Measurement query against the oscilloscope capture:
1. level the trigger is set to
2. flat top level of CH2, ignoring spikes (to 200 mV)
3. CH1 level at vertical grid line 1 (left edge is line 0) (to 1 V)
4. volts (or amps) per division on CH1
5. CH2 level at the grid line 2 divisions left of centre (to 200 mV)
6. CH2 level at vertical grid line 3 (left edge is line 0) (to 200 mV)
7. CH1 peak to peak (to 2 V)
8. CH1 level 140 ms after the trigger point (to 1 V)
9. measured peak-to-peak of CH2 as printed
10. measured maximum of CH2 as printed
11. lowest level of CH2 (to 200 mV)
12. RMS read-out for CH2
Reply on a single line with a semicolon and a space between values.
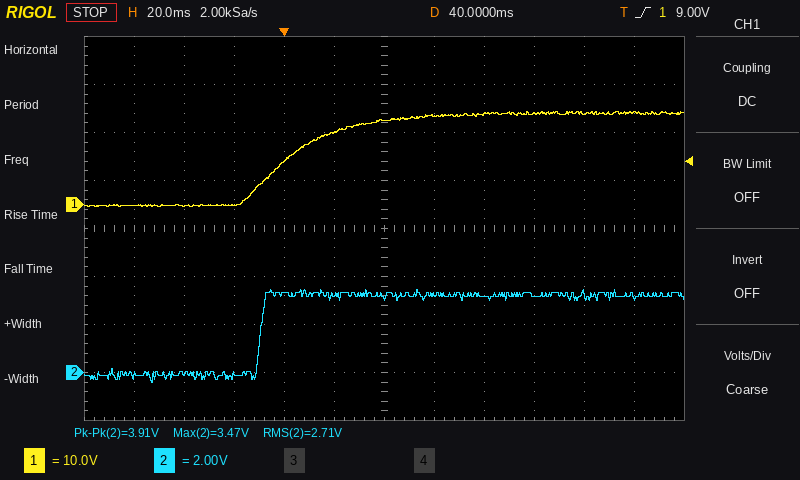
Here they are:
9.00 V; 3.2 V; 0 V; 10 V; 3.2 V; -200 mV; 20 V; 19 V; 3.91 V; 3.47 V; -400 mV; 2.71 V
